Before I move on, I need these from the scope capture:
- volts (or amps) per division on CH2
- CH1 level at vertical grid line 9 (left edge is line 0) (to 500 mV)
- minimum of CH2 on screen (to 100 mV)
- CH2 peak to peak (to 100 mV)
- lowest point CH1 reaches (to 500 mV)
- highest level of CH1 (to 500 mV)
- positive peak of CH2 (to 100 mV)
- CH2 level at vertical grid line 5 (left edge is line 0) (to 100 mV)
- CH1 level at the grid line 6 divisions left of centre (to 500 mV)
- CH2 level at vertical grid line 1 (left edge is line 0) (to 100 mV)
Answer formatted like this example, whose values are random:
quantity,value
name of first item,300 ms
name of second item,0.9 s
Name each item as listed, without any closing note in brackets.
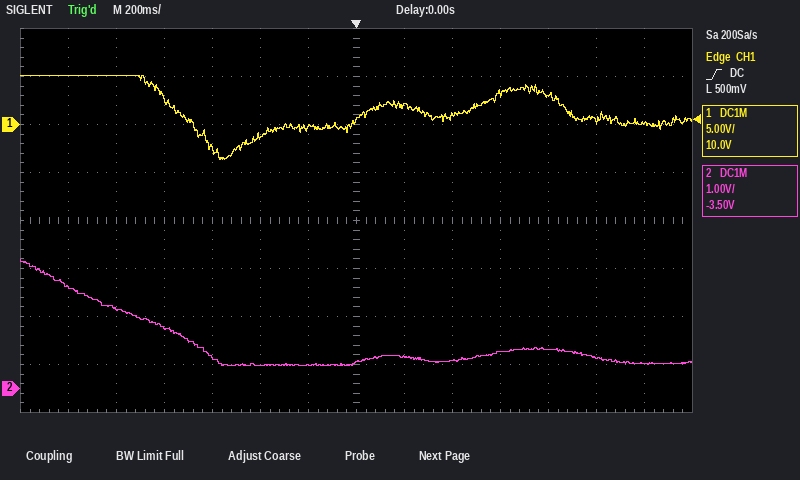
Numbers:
quantity,value
volts (or amps) per division on CH2,1 V
CH1 level at vertical grid line 9 (left edge is line 0),1.0 V
minimum of CH2 on screen,500 mV
CH2 peak to peak,2.2 V
lowest point CH1 reaches,-3.5 V
highest level of CH1,5.0 V
positive peak of CH2,2.7 V
CH2 level at vertical grid line 5 (left edge is line 0),500 mV
CH1 level at the grid line 6 divisions left of centre,5.0 V
CH2 level at vertical grid line 1 (left edge is line 0),2.1 V
